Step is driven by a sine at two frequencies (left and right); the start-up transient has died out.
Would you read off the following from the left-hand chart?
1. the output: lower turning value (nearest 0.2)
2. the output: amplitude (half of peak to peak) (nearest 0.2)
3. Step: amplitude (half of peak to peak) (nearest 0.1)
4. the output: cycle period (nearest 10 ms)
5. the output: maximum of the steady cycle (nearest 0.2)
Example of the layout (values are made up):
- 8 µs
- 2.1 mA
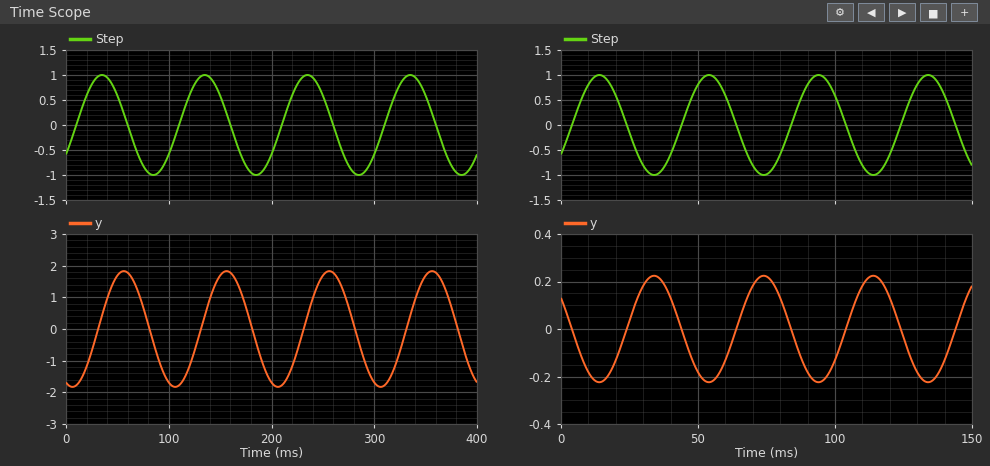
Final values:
- -1.8
- 1.8
- 1.0
- 100 ms
- 1.8
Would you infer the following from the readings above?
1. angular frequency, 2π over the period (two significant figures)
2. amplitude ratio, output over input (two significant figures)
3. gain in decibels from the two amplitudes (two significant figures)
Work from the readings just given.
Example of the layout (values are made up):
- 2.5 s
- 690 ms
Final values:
- 0.063 rad/ms
- 1.8
- 5.1 dB
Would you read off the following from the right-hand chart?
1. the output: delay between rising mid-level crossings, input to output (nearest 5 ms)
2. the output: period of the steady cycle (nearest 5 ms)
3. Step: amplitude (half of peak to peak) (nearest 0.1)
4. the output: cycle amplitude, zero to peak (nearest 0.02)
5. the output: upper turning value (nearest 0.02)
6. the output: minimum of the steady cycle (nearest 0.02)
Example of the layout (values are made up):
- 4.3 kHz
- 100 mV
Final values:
- 20 ms
- 40 ms
- 1.0
- 0.22
- 0.22
- -0.22
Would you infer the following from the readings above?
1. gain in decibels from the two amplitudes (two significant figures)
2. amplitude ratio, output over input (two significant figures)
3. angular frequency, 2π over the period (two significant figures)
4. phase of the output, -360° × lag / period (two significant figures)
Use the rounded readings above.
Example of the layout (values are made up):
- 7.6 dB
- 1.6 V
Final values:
- -13 dB
- 0.22
- 0.16 rad/ms
- -180°
